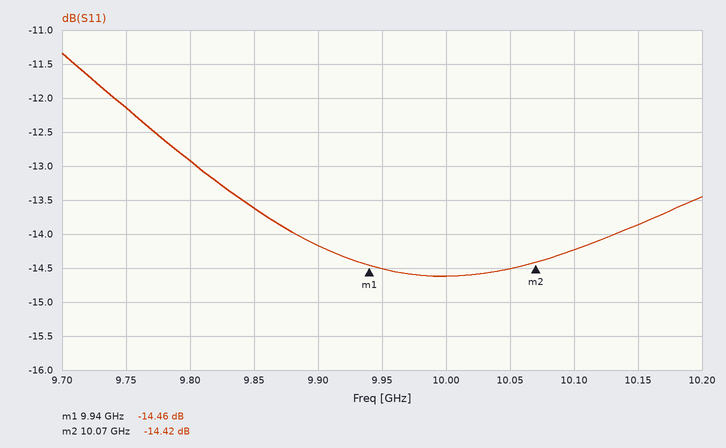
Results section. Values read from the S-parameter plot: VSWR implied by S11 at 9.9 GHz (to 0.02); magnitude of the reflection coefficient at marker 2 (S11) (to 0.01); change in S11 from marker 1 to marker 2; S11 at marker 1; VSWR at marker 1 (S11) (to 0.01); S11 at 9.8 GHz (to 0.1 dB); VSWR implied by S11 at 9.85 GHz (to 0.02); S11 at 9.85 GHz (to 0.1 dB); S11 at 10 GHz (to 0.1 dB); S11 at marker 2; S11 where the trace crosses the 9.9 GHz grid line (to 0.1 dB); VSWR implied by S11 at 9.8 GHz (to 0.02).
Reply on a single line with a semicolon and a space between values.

1.48; 0.19; 0.04 dB; -14.46 dB; 1.47; -12.9 dB; 1.52; -13.6 dB; -14.6 dB; -14.42 dB; -14.2 dB; 1.58
